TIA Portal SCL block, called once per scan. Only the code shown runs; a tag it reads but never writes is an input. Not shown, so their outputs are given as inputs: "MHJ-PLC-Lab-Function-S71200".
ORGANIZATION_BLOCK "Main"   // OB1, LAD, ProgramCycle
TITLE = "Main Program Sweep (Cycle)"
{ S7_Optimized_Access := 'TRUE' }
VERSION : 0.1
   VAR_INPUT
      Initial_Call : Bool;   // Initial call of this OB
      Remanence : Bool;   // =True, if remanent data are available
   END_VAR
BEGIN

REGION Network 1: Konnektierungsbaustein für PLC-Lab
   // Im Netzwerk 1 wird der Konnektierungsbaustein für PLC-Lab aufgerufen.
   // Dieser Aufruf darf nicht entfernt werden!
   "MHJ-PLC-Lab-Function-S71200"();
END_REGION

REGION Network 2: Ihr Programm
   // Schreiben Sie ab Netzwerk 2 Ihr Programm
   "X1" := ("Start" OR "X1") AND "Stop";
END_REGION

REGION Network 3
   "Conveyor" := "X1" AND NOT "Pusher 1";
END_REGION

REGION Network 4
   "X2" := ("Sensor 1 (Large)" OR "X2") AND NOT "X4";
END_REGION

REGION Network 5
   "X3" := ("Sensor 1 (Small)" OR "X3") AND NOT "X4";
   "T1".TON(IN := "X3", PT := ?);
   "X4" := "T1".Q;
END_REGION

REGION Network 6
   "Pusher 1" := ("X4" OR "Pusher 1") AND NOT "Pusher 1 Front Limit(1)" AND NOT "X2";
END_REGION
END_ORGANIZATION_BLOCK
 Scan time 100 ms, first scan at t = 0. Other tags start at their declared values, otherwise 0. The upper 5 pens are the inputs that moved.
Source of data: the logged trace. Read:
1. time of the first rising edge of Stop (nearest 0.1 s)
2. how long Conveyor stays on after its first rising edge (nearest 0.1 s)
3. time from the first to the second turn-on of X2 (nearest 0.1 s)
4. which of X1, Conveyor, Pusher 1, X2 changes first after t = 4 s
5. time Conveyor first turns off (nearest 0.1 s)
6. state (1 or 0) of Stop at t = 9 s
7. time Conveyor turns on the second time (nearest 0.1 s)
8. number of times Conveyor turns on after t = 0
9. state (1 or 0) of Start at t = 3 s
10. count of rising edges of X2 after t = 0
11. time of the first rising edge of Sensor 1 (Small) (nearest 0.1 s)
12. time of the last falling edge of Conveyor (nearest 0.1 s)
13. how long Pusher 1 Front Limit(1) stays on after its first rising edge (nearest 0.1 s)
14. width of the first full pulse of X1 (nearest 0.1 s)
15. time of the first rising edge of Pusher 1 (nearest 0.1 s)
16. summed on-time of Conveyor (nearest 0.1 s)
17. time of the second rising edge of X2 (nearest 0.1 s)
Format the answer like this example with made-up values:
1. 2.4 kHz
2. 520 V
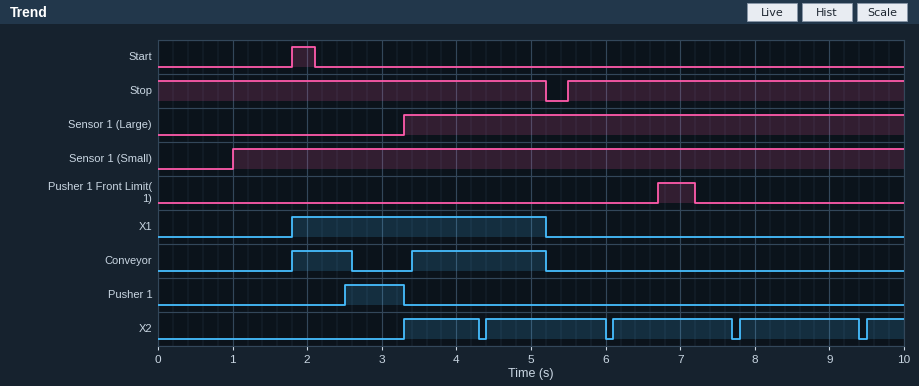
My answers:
1. 5.5 s
2. 0.8 s
3. 1.1 s
4. X2
5. 2.6 s
6. 1
7. 3.4 s
8. 2
9. 0
10. 5
11. 1.0 s
12. 5.2 s
13. 0.5 s
14. 3.4 s
15. 2.5 s
16. 2.6 s
17. 4.4 s
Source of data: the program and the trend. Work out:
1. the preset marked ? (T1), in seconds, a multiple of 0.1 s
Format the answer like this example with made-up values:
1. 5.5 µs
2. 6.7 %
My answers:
1. 1.5 s
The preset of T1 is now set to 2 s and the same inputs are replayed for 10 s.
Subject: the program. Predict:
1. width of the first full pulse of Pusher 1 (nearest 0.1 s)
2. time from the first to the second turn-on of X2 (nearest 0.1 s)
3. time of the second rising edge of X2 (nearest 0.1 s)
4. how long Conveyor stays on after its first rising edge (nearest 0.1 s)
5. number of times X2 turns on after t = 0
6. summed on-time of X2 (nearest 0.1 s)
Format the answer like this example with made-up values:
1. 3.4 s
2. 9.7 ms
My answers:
1. 0.3 s
2. 2.1 s
3. 5.4 s
4. 1.3 s
5. 4
6. 6.4 s
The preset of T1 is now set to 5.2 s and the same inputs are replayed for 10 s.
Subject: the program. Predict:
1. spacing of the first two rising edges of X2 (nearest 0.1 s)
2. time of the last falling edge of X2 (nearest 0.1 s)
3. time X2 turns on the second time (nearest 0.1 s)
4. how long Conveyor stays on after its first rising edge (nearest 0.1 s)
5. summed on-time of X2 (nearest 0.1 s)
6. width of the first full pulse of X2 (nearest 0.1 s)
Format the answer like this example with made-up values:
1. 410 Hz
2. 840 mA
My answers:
1. 3.1 s
2. 6.3 s
3. 6.4 s
4. 3.4 s
5. 6.6 s
6. 3.0 s
